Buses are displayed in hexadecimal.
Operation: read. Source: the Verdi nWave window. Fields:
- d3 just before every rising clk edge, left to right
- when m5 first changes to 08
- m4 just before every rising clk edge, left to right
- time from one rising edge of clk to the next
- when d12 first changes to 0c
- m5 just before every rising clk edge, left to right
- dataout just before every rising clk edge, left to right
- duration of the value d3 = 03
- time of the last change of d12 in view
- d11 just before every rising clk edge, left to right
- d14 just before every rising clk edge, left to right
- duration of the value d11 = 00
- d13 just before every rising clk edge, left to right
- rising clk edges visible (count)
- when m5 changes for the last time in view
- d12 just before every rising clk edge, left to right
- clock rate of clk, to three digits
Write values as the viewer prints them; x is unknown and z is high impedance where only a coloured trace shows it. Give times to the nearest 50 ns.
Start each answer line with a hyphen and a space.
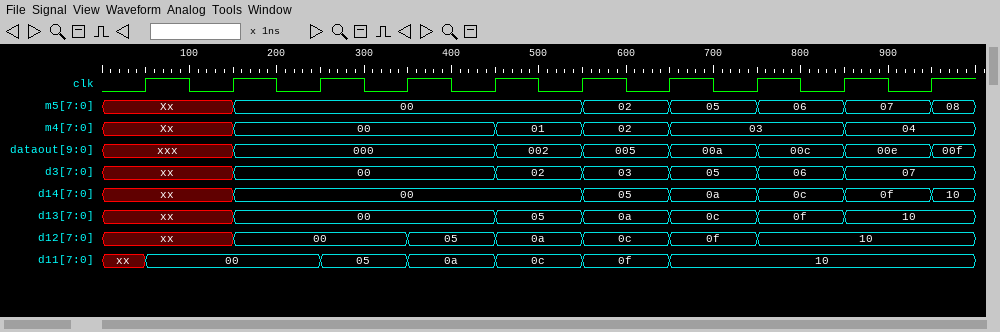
- xx, xx, 00, 00, 00, 02, 03, 05, 06, 07
- 950 ns
- Xx, Xx, 00, 00, 00, 01, 02, 03, 03, 04
- 100 ns
- 550 ns
- Xx, Xx, 00, 00, 00, 00, 02, 05, 06, 07
- xxx, xxx, 000, 000, 000, 002, 005, 00a, 00c, 00e
- 100 ns
- 750 ns
- xx, 00, 00, 05, 0a, 0c, 0f, 10, 10, 10
- xx, xx, 00, 00, 00, 00, 05, 0a, 0c, 0f
- 200 ns
- xx, xx, 00, 00, 00, 05, 0a, 0c, 0f, 10
- 10
- 950 ns
- xx, xx, 00, 00, 05, 0a, 0c, 0f, 10, 10
- 10.0 MHz
